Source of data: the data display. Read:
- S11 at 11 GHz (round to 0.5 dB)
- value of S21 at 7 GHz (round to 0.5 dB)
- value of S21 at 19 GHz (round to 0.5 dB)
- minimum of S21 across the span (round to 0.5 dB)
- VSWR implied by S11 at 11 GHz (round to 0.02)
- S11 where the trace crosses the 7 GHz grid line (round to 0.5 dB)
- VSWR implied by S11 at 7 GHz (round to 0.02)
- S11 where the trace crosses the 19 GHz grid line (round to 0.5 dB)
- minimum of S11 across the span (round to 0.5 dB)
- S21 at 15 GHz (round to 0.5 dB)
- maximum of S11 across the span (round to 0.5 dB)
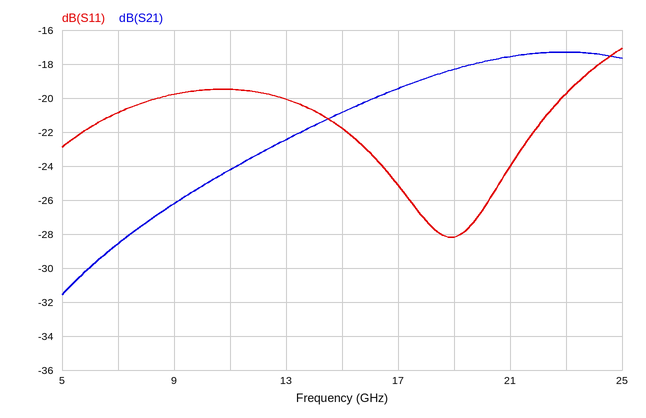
-19.5 dB
-28.5 dB
-18.5 dB
-31.5 dB
1.24
-21.0 dB
1.20
-28.0 dB
-28.0 dB
-21.0 dB
-17.0 dB
